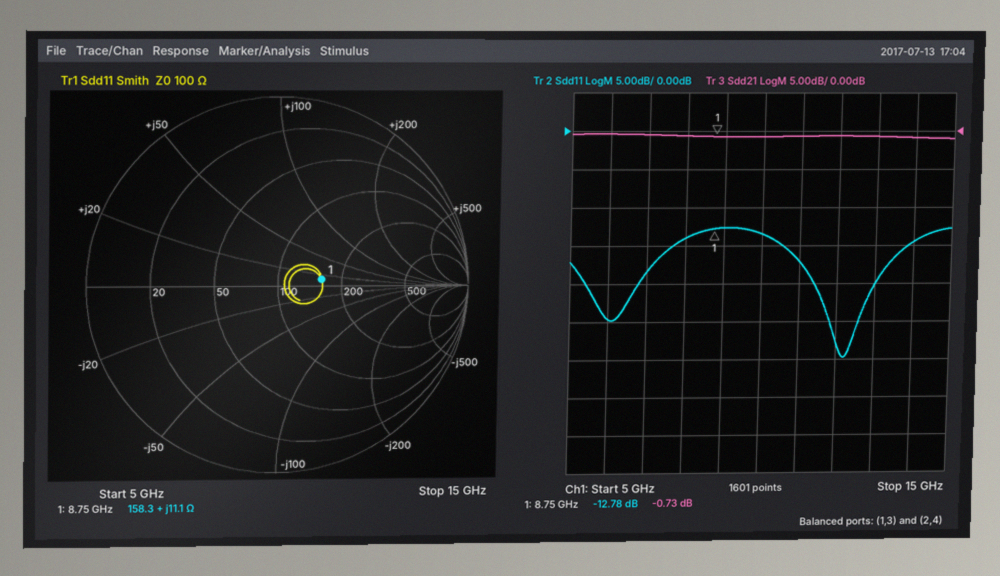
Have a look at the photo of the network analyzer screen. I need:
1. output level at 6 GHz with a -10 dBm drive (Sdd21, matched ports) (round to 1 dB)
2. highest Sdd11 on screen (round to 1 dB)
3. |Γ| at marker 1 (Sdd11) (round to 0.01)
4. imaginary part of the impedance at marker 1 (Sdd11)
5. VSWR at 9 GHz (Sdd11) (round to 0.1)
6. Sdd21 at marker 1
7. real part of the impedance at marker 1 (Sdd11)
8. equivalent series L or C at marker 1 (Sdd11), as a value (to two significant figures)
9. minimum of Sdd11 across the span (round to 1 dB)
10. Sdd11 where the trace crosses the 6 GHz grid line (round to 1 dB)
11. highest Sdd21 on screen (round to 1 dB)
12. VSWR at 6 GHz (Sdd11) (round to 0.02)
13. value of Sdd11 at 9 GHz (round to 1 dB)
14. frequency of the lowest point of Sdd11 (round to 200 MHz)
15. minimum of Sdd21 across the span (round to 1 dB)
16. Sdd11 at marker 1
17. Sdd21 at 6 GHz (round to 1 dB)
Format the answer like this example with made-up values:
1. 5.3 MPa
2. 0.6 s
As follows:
1. -10 dBm
2. -13 dB
3. 0.23
4. +11.1 Ω
5. 1.6
6. -0.73 dB
7. 158.3 Ω
8. 200 pH
9. -30 dB
10. -25 dB
11. 0 dB
12. 1.12
13. -13 dB
14. 12.2 GHz
15. -1 dB
16. -12.78 dB
17. 0 dB
